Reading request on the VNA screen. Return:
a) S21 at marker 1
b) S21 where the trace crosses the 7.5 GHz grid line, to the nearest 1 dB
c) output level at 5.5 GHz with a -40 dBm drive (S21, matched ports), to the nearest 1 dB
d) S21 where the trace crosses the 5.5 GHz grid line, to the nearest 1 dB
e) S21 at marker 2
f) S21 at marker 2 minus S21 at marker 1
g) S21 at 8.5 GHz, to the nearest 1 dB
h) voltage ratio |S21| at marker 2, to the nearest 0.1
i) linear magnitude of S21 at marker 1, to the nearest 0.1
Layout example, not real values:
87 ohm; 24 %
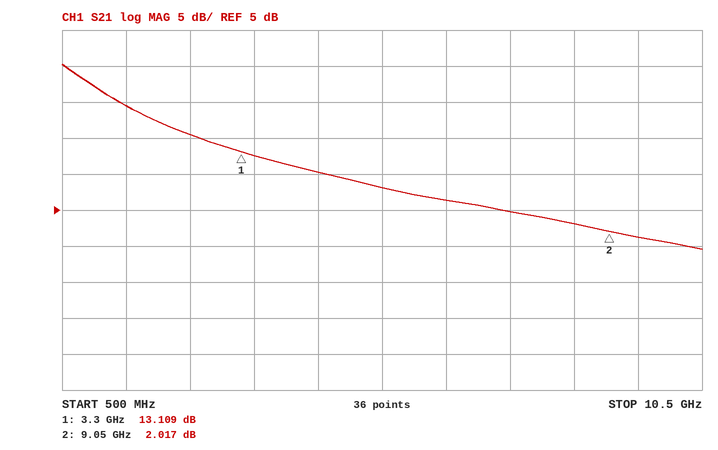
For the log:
13.109 dB; 5 dB; -32 dBm; 8 dB; 2.017 dB; -11.092 dB; 3 dB; 1.3; 4.5
